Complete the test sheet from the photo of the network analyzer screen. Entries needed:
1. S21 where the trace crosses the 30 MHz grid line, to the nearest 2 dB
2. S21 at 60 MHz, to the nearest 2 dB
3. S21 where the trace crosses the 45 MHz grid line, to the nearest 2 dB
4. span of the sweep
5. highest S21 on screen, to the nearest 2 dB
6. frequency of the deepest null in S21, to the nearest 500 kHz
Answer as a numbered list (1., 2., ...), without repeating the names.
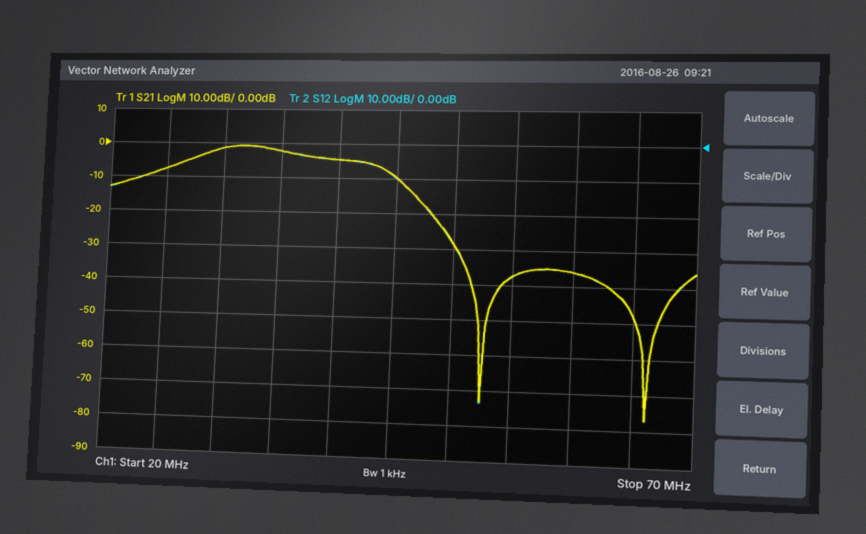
1. -2 dB
2. -36 dB
3. -10 dB
4. 50 MHz
5. 0 dB
6. 66.0 MHz
